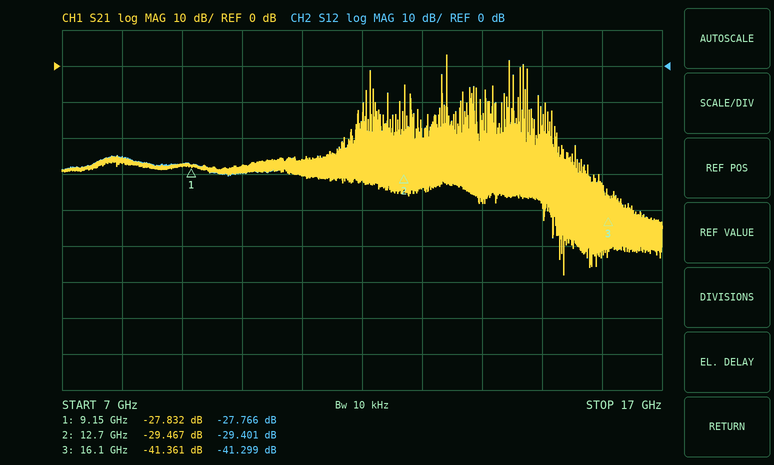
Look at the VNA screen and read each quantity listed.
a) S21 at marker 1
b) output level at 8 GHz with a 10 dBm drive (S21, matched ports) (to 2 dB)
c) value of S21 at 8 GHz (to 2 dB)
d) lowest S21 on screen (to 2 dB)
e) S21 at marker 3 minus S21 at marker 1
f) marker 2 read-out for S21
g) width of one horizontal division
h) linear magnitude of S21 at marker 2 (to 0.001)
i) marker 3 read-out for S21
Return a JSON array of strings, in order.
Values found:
["-27.832 dB", "-16 dBm", "-26 dB", "-58 dB", "-13.529 dB", "-29.467 dB", "1 GHz", "0.034", "-41.361 dB"]
